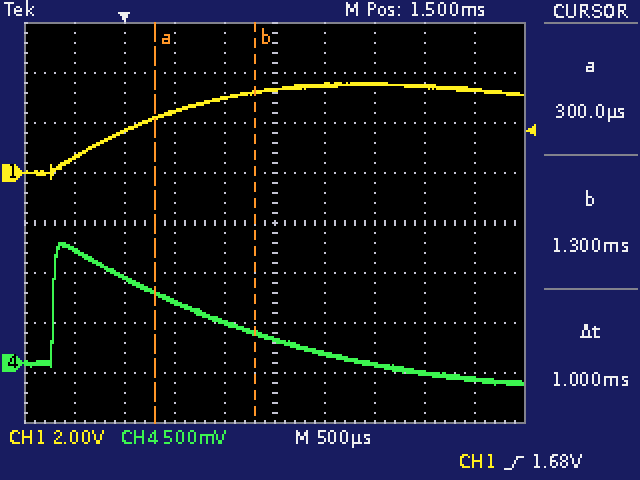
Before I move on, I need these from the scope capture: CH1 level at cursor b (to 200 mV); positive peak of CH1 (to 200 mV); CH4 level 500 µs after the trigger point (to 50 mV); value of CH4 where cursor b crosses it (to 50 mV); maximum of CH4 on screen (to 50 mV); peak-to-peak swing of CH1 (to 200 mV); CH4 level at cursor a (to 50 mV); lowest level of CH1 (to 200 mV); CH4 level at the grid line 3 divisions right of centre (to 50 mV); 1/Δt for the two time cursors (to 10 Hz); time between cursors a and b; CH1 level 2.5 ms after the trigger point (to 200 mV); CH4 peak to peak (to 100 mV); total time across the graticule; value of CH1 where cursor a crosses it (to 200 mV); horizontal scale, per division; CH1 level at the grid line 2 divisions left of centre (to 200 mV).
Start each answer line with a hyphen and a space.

- 3.2 V
- 3.6 V
- 600 mV
- 300 mV
- 1.20 V
- 3.8 V
- 700 mV
- -200 mV
- -100 mV
- 1.00 kHz
- 1 ms
- 3.6 V
- 1.40 V
- 5 ms
- 2.2 V
- 500 µs
- 2.4 V
